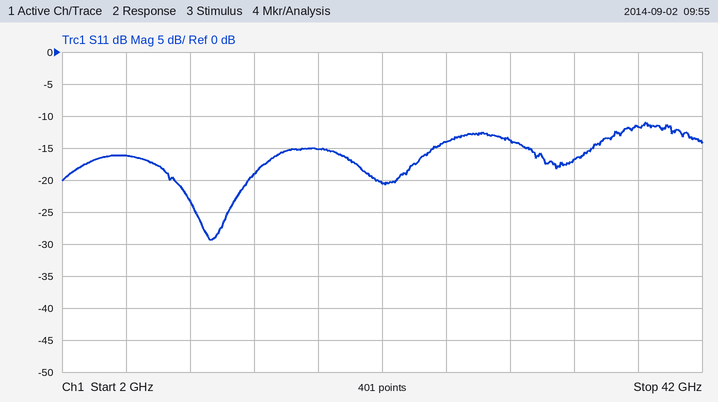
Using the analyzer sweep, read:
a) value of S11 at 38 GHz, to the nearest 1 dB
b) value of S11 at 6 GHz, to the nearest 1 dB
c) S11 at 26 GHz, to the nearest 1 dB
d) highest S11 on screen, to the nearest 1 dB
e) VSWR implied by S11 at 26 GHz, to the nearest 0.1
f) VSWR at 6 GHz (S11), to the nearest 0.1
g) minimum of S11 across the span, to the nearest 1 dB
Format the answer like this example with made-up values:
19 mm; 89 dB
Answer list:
-12 dB; -16 dB; -14 dB; -11 dB; 1.5; 1.4; -29 dB
